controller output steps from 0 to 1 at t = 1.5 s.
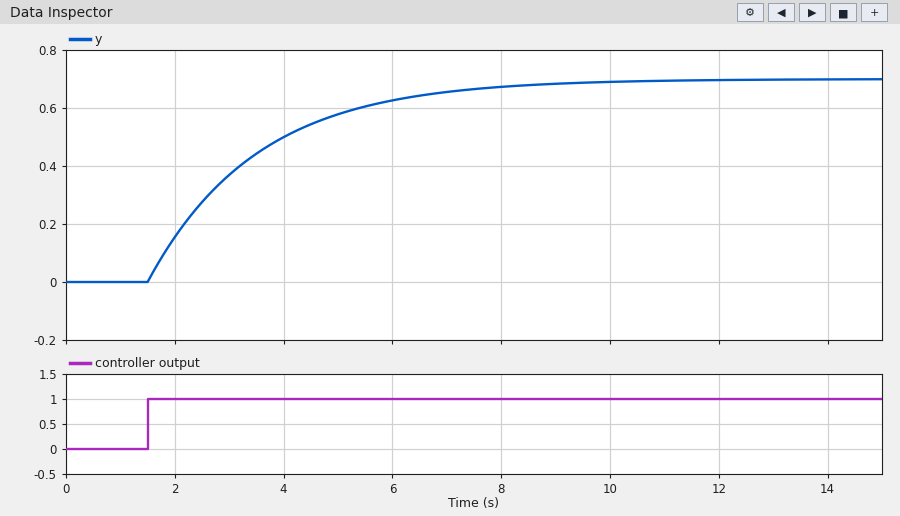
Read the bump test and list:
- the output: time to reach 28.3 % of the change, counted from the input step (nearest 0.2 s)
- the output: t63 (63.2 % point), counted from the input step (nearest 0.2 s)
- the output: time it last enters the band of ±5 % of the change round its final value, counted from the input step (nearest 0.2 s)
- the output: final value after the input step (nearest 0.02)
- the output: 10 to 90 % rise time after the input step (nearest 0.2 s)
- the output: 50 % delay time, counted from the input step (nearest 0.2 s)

0.6 s
2.0 s
6.0 s
0.70
4.4 s
1.4 s
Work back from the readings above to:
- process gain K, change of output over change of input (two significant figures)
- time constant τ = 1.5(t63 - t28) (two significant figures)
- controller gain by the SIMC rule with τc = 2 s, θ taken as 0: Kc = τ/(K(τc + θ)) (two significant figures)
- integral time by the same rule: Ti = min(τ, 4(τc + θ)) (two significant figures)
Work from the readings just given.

0.70
2.1 s
1.5
2.1 s
